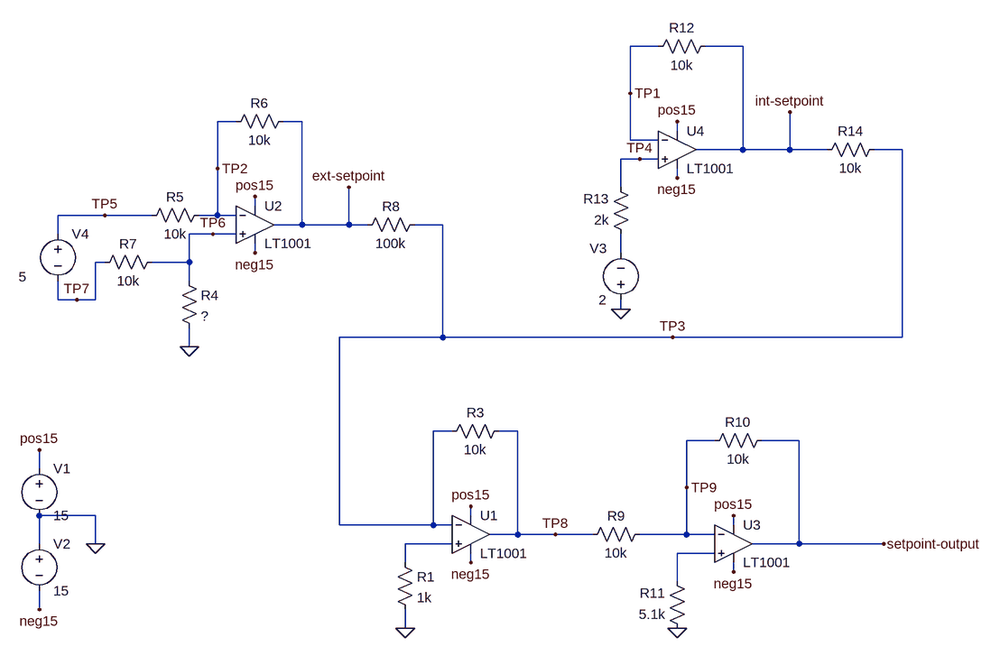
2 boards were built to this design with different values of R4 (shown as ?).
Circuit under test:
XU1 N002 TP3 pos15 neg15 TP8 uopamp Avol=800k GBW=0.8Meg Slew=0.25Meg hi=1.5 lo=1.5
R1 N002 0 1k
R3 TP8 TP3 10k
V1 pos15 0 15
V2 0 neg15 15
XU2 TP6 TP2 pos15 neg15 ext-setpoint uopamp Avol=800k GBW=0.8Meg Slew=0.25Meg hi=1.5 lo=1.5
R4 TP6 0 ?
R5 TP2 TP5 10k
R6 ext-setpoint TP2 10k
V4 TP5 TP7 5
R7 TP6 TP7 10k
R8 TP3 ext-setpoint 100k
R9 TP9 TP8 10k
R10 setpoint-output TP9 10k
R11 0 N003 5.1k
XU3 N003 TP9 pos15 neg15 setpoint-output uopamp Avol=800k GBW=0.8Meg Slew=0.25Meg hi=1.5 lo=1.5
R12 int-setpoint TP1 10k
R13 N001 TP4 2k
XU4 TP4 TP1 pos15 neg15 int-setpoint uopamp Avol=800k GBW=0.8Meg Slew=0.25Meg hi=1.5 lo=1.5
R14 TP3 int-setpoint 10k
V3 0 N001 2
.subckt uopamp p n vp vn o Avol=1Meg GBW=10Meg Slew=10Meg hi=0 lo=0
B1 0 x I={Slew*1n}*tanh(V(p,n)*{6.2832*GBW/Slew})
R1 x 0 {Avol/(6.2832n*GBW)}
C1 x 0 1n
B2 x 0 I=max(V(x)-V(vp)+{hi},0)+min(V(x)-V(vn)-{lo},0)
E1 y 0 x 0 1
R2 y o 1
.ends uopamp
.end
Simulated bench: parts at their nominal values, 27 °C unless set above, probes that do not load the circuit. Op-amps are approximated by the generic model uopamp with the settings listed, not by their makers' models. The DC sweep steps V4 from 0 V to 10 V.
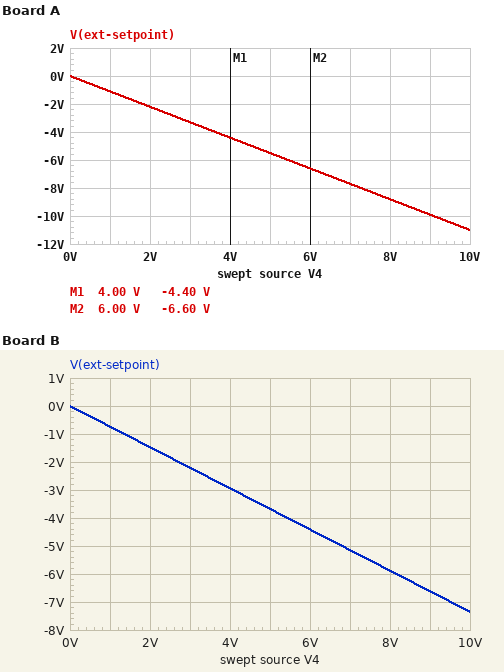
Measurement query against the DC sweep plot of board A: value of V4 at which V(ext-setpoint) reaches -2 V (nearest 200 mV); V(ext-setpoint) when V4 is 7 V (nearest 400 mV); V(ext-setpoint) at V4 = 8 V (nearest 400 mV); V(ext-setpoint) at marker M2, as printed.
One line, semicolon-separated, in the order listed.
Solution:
1.8 V; -7.6 V; -8.8 V; -6.60 V
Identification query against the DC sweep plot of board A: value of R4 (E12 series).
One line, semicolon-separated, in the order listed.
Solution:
12 kΩ
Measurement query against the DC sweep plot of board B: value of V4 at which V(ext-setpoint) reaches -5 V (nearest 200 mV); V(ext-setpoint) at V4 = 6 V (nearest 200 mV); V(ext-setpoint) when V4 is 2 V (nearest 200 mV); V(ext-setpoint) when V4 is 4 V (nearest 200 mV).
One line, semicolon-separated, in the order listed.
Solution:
6.8 V; -4.4 V; -1.4 V; -3.0 V
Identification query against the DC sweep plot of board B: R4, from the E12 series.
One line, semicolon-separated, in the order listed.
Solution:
4.7 kΩ
